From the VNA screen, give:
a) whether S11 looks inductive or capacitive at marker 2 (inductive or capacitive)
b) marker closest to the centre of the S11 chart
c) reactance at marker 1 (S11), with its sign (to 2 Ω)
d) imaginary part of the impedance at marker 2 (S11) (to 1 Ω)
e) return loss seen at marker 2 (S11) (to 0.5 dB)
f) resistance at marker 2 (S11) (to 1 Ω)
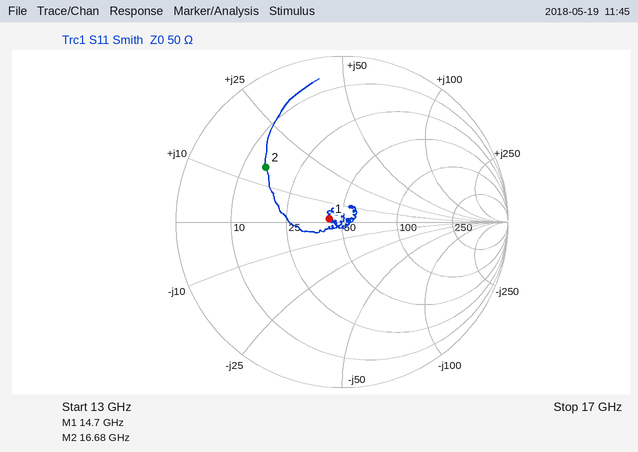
inductive
marker 1
+2 Ω
+15 Ω
5.0 dB
15 Ω
